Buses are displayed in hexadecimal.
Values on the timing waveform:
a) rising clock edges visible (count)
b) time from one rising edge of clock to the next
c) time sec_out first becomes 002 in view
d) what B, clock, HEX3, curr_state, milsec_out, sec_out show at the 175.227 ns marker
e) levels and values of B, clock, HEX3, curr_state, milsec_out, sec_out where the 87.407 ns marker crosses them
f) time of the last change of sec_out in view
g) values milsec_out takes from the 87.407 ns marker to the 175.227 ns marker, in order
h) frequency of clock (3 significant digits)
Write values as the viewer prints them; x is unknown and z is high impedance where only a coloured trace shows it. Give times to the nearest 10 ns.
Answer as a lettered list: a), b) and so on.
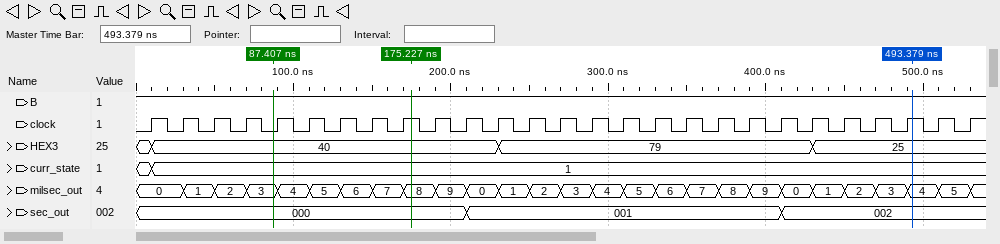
a) 27
b) 20 ns
c) 410 ns
d) B=1, clock=1, HEX3=40, curr_state=1, milsec_out=8, sec_out=000
e) B=1, clock=0, HEX3=40, curr_state=1, milsec_out=3, sec_out=000
f) 410 ns
g) 3, 4, 5, 6, 7, 8
h) 50.0 MHz
